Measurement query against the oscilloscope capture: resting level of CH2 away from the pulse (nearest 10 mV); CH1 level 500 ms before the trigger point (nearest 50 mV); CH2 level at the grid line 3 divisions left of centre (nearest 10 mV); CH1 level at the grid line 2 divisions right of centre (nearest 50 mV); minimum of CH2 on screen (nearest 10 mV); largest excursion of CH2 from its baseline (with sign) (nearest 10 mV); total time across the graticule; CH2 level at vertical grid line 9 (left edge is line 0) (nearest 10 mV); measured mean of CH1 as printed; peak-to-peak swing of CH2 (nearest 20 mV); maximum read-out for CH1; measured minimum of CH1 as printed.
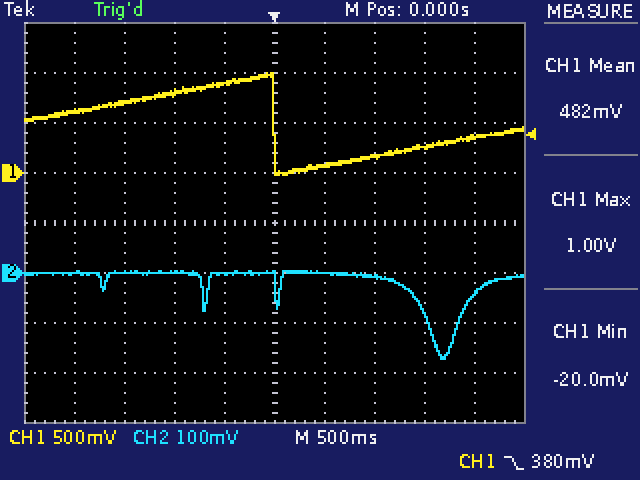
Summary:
0 mV
900 mV
0 mV
150 mV
-170 mV
-170 mV
5 s
-40 mV
482 mV
180 mV
1.00 V
-20.0 mV
